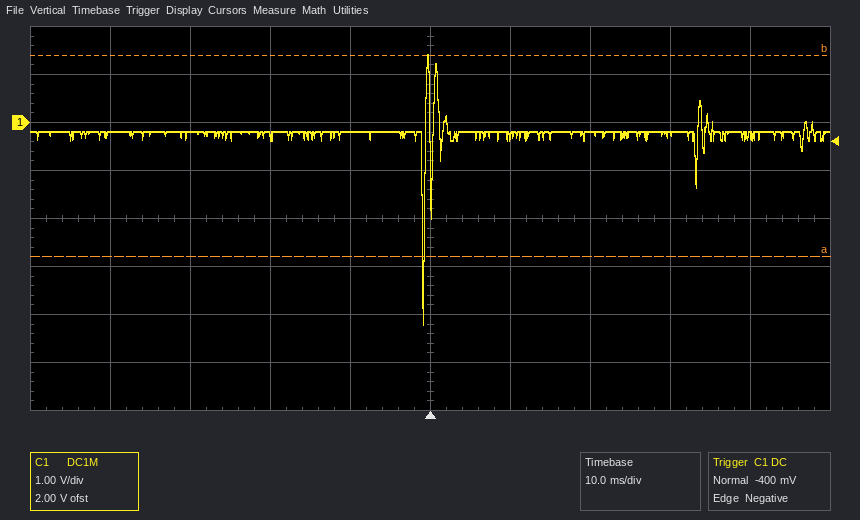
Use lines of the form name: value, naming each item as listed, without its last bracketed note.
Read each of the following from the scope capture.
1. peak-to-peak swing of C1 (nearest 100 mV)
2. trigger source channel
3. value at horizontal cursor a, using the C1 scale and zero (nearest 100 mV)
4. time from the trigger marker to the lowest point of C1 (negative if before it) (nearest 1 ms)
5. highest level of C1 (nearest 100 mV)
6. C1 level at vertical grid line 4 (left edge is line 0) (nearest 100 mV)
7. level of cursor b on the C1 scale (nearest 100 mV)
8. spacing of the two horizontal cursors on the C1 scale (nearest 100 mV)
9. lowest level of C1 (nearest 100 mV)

peak-to-peak swing of C1: 5.6 V
trigger source channel: C1
value at horizontal cursor a, using the C1 scale and zero: -2.8 V
time from the trigger marker to the lowest point of C1 (negative if before it): -1 ms
highest level of C1: 1.4 V
C1 level at vertical grid line 4 (left edge is line 0): -200 mV
level of cursor b on the C1 scale: 1.4 V
spacing of the two horizontal cursors on the C1 scale: 4.2 V
lowest level of C1: -4.2 V
